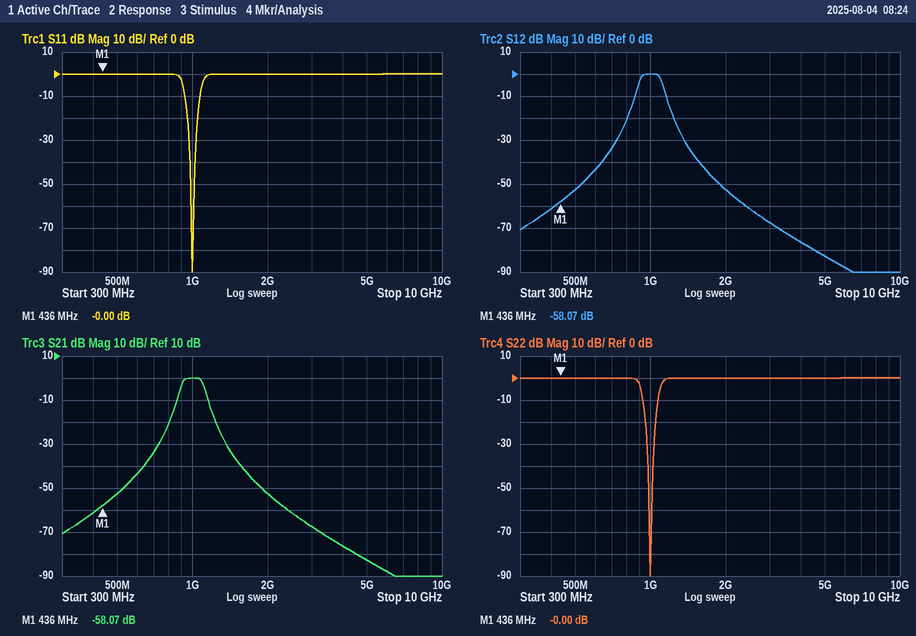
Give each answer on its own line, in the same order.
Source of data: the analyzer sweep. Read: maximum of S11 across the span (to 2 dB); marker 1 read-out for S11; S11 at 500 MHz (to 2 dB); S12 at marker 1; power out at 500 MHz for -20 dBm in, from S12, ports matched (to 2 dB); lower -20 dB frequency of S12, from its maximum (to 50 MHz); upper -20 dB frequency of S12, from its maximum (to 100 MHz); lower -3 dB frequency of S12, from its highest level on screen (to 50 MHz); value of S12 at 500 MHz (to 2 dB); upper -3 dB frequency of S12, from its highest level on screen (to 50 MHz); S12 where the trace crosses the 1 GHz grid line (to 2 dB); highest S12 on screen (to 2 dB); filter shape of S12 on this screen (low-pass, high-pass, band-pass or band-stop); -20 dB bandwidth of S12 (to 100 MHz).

0 dB
-0.00 dB
0 dB
-58.07 dB
-72 dBm
800 MHz
1.2 GHz
900 MHz
-52 dB
1.10 GHz
0 dB
0 dB
band-pass
400 MHz
